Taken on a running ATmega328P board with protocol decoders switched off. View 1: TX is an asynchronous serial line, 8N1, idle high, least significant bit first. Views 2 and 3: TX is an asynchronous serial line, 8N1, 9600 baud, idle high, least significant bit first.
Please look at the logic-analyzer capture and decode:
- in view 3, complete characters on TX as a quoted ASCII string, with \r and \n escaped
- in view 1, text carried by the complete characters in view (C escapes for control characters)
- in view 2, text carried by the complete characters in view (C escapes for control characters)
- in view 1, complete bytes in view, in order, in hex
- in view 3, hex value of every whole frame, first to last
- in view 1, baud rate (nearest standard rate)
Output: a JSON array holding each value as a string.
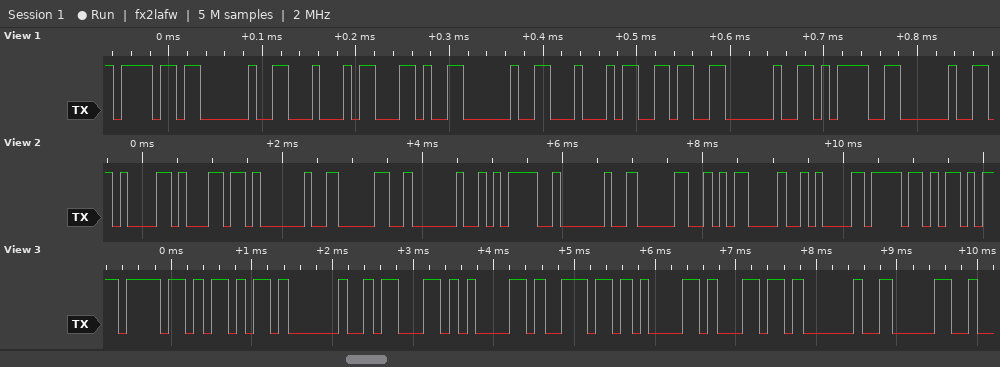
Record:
["\"ok canal 0\"", "\"o D, D6 = \"", "\"al 0 = 0\\r\\no\"", "6F 20 44 2C 20 44 36 20 3D 20", "6F 6B 20 63 61 6E 61 6C 20 30", "115200 baud"]
